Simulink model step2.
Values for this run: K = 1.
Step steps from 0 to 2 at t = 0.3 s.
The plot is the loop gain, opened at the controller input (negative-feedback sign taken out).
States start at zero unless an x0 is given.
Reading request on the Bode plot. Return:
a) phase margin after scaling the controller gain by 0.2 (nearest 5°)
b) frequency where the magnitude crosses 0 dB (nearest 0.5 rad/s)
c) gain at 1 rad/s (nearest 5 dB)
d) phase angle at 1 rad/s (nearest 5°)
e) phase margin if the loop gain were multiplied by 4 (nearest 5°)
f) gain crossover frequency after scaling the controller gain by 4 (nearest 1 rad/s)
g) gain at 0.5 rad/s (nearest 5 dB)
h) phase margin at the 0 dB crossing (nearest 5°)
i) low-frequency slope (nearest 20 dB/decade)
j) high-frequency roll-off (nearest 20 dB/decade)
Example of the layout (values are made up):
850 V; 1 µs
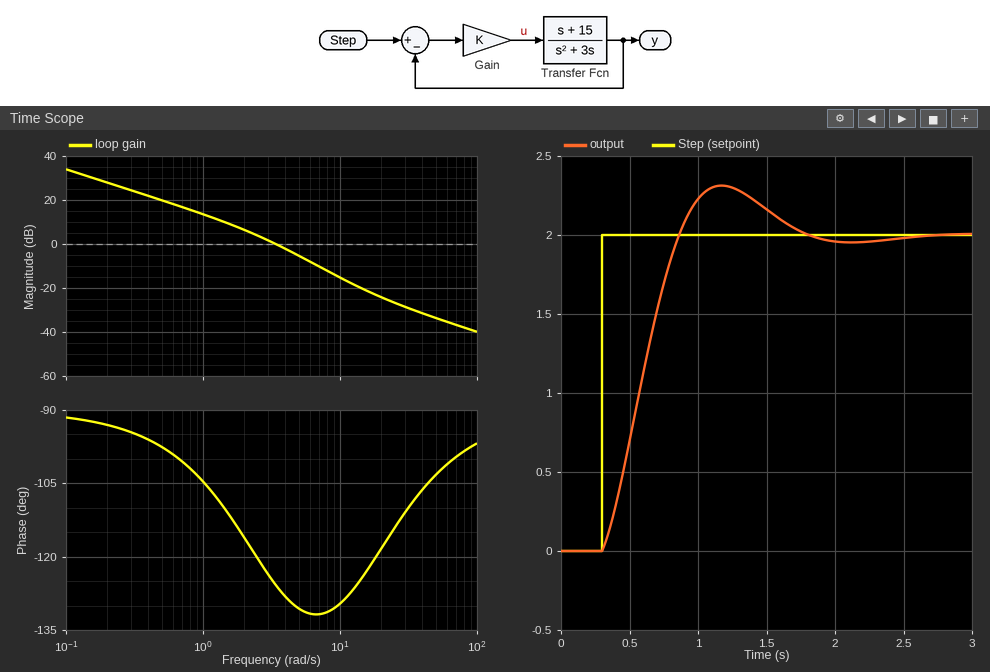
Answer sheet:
75°; 3.5 rad/s; 15 dB; -105°; 50°; 8 rad/s; 20 dB; 55°; -20 dB/decade; -20 dB/decade
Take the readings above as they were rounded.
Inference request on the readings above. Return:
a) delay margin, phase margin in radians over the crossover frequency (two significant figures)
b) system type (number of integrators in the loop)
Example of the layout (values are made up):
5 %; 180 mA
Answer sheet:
0.27 s; 1
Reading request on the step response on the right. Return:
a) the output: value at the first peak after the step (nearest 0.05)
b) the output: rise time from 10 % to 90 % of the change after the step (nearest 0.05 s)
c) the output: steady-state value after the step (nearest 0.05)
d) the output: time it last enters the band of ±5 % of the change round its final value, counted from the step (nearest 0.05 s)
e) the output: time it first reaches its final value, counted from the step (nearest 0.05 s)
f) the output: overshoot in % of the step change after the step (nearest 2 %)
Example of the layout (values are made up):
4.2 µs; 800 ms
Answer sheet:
2.30; 0.40 s; 2.00; 1.30 s; 0.55 s; 16 %
